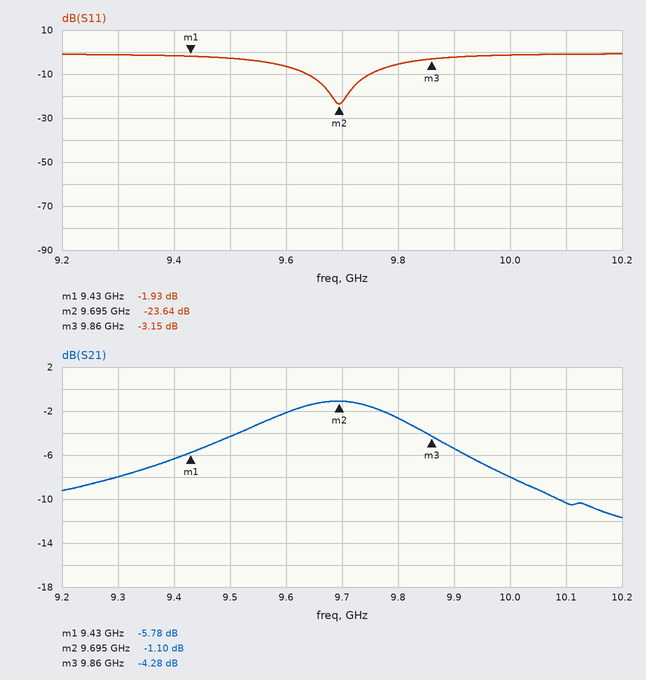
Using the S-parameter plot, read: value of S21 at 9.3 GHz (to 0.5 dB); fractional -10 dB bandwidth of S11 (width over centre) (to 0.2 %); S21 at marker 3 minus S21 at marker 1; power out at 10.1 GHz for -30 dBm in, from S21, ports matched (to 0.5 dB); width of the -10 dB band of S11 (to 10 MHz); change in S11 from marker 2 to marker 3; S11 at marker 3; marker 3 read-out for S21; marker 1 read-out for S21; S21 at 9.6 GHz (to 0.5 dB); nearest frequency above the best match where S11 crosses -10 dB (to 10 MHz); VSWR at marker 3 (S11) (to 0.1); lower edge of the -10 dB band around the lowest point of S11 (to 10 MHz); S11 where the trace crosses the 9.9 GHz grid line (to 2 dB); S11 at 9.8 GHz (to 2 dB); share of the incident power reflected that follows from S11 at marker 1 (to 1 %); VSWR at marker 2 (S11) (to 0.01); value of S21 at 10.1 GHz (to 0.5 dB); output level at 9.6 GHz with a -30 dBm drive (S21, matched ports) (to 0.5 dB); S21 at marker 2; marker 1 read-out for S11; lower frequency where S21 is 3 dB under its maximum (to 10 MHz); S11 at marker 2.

-8.0 dB
1.2 %
1.50 dB
-40.5 dBm
110 MHz
20.49 dB
-3.15 dB
-4.28 dB
-5.78 dB
-2.0 dB
9.75 GHz
5.6
9.64 GHz
-2 dB
-6 dB
64 %
1.14
-10.5 dB
-32.0 dBm
-1.10 dB
-1.93 dB
9.51 GHz
-23.64 dB
